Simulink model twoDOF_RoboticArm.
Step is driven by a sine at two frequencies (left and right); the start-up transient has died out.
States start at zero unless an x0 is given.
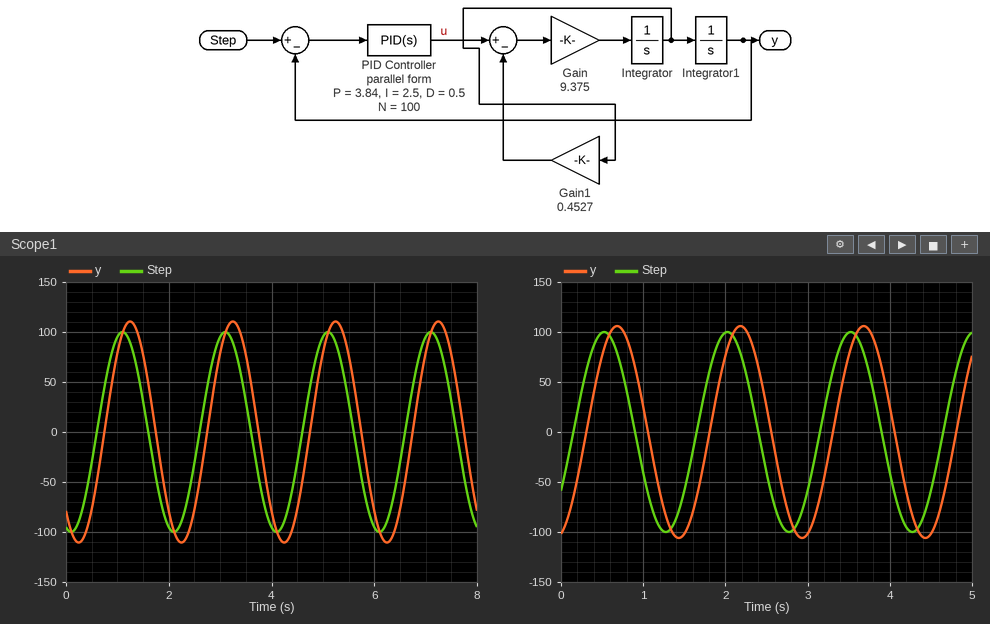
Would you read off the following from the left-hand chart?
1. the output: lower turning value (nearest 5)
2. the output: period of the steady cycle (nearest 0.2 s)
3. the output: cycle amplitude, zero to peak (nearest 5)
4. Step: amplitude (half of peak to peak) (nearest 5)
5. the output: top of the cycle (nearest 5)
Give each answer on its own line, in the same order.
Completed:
-110
2.0 s
110
100
110
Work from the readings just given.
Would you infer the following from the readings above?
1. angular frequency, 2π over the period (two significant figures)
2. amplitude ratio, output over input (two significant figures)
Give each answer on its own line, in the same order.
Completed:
3.1 rad/s
1.1
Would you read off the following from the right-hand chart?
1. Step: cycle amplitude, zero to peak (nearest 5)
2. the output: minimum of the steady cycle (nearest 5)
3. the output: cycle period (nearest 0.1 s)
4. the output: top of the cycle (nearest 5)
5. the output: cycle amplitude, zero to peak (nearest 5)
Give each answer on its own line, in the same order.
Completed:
100
-105
1.5 s
105
105
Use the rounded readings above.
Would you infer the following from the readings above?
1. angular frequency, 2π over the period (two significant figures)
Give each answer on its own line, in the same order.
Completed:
4.2 rad/s
